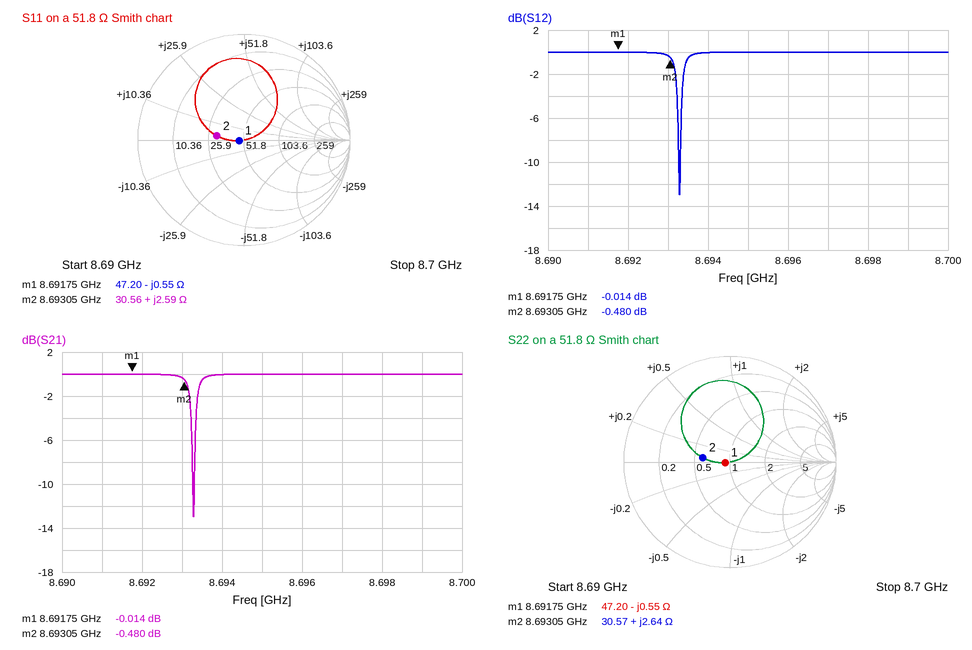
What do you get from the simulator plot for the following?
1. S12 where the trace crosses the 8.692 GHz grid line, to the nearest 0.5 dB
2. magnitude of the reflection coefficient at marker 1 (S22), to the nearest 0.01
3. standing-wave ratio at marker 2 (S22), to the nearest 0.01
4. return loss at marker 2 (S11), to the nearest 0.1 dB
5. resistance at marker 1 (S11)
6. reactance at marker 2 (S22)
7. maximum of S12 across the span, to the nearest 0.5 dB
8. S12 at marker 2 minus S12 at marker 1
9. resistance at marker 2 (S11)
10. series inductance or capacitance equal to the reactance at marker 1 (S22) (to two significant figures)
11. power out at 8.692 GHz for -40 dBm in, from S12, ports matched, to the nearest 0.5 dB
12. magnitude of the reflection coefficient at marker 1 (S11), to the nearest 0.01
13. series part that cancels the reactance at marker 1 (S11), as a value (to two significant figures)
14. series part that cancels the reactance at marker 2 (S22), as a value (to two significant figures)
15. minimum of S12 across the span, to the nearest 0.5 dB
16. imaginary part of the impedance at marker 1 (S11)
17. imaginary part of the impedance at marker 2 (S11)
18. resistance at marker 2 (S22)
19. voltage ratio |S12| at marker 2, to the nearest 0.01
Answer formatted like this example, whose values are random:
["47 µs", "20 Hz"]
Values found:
["0.0 dB", "0.05", "1.70", "11.7 dB", "47.20 Ω", "+2.64 Ω", "0.0 dB", "-0.466 dB", "30.56 Ω", "33 pF", "-40.0 dBm", "0.05", "10 pH", "6.9 pF", "-13.0 dB", "-0.55 Ω", "+2.59 Ω", "30.57 Ω", "0.95"]
